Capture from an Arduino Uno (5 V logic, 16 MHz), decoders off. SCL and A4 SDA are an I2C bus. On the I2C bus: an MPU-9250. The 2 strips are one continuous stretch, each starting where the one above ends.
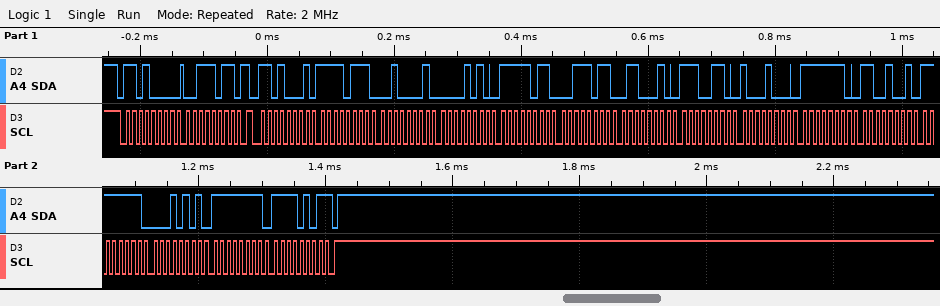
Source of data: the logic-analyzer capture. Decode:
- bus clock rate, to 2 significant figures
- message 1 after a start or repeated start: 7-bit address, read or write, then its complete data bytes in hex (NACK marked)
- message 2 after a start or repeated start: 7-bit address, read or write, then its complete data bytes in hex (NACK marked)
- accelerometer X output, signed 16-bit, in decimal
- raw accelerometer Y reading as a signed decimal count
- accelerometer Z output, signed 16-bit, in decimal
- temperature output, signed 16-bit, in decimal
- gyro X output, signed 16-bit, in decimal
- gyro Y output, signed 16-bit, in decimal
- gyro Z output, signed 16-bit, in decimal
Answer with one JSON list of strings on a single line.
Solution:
["100 kHz", "0x68 write: 3B", "0x68 read: F7 21 0A FB 3B 62 E6 88 FE C9 FF 15 FF F5 NACK", "-2271", "2811", "15202", "-6520", "-311", "-235", "-11"]
